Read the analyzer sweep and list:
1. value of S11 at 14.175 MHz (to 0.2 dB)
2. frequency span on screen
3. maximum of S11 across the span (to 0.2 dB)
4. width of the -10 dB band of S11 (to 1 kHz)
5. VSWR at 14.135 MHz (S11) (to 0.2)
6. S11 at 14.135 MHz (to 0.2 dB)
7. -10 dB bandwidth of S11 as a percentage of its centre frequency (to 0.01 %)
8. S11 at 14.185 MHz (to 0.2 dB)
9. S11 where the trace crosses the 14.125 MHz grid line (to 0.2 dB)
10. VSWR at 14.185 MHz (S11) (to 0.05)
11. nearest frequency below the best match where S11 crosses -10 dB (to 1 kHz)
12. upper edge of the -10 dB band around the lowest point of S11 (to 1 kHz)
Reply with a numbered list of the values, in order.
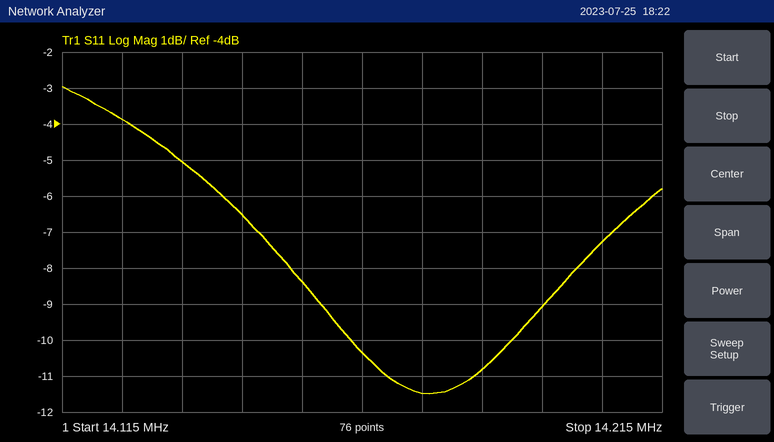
1. -11.4 dB
2. 100 kHz
3. -3.0 dB
4. 27 kHz
5. 3.6
6. -5.0 dB
7. 0.19 %
8. -10.8 dB
9. -3.8 dB
10. 1.80
11. 14.163 MHz
12. 14.190 MHz
